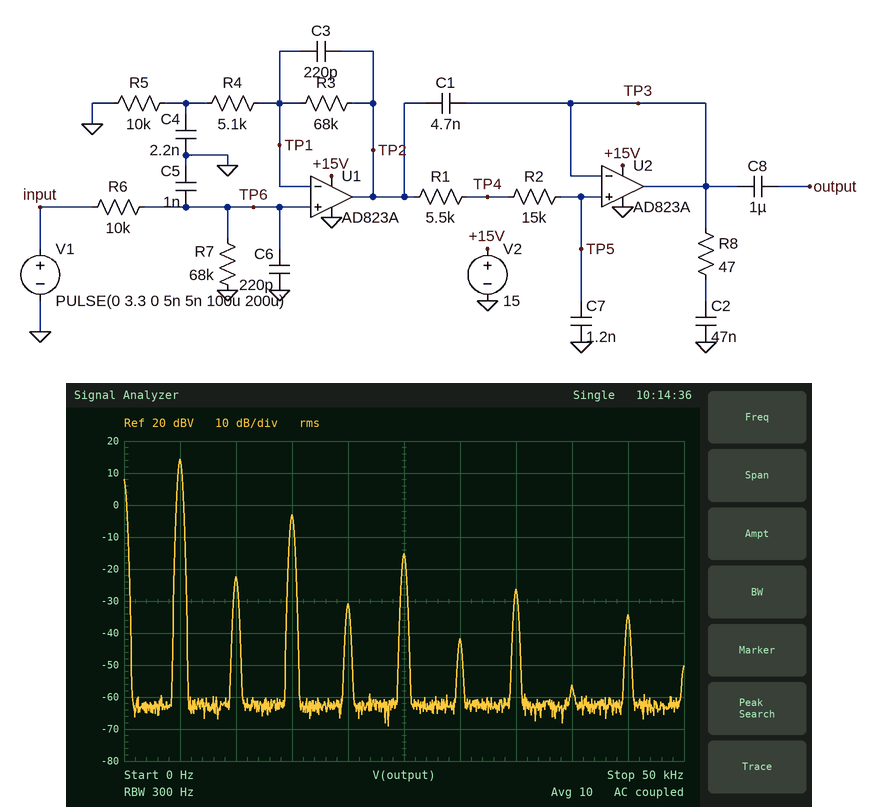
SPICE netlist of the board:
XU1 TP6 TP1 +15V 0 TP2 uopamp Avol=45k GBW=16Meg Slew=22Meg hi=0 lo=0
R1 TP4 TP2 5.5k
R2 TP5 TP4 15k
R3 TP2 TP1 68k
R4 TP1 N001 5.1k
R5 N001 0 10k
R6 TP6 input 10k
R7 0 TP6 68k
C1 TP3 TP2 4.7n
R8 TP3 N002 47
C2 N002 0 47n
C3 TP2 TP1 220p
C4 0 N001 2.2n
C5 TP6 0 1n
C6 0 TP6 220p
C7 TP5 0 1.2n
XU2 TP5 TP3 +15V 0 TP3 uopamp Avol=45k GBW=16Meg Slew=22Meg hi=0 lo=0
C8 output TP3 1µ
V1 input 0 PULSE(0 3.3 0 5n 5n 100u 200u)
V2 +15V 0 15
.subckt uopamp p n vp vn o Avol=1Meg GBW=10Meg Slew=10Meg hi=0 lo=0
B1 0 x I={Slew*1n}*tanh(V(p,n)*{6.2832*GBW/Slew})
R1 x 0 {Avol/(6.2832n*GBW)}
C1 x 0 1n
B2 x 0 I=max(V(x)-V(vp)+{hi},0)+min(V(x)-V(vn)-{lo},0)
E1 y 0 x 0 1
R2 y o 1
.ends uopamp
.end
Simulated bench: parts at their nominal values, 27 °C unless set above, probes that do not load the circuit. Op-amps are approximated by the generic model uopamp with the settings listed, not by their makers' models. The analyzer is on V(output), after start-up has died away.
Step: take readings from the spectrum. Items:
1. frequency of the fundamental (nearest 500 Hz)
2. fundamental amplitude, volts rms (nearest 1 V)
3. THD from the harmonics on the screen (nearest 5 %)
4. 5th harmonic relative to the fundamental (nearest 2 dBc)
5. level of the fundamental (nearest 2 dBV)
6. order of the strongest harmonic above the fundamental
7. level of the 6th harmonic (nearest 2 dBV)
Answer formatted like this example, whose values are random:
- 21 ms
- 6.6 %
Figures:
- 5.0 kHz
- 5 V
- 15 %
- -30 dBc
- 14 dBV
- 3
- -42 dBV
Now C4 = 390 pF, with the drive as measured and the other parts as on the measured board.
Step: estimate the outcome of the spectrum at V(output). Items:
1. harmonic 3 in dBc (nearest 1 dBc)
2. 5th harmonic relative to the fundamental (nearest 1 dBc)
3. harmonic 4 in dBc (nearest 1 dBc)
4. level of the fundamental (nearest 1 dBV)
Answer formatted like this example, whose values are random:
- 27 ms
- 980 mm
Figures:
- -21 dBc
- -34 dBc
- -56 dBc
- 14 dBV
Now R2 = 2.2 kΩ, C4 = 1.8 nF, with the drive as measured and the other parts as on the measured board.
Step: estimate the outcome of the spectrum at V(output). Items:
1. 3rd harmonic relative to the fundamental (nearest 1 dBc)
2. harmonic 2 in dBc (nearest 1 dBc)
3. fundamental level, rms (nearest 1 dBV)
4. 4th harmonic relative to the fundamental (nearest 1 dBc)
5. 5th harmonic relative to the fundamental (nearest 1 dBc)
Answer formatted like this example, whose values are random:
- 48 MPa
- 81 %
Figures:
- -14 dBc
- -33 dBc
- 16 dBV
- -42 dBc
- -25 dBc
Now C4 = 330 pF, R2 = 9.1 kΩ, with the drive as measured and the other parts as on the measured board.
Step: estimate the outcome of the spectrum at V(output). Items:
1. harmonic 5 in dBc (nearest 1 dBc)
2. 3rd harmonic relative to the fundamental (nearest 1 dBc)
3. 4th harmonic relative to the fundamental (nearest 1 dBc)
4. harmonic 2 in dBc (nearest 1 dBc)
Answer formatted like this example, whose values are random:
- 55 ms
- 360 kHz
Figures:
- -33 dBc
- -20 dBc
- -54 dBc
- -36 dBc
